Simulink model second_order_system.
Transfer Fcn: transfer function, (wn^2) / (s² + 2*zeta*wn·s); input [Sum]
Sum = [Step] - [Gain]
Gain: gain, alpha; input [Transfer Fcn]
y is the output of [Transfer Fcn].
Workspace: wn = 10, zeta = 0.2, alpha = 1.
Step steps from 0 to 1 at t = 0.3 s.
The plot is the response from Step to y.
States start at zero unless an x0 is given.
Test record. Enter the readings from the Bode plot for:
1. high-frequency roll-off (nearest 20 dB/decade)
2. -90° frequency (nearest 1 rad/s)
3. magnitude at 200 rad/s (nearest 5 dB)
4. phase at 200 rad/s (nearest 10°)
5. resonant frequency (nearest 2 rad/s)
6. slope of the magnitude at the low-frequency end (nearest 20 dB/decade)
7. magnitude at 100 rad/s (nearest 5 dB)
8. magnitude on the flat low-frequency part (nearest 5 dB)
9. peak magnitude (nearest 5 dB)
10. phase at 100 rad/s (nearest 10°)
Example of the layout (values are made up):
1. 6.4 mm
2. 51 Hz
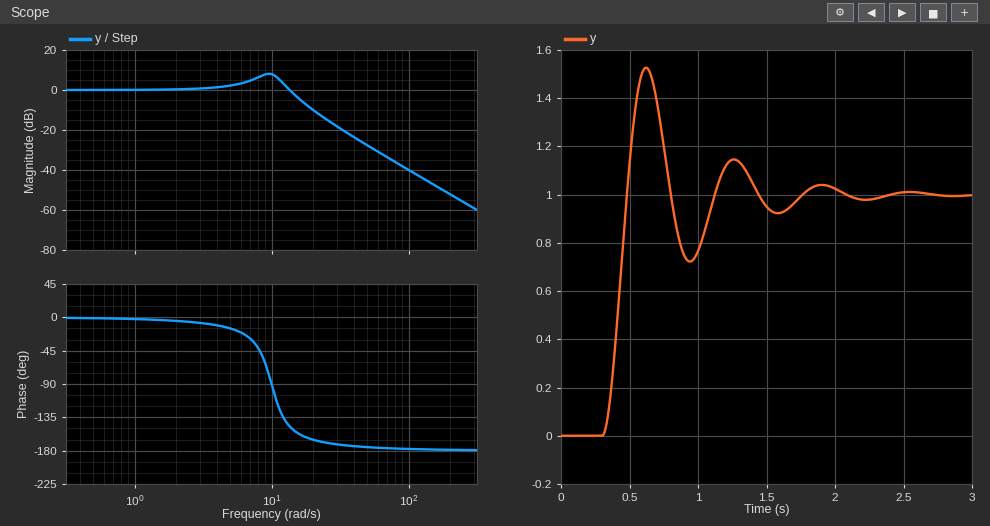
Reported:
1. -40 dB/decade
2. 10 rad/s
3. -50 dB
4. -180°
5. 10 rad/s
6. 0 dB/decade
7. -40 dB
8. 0 dB
9. 10 dB
10. -180°
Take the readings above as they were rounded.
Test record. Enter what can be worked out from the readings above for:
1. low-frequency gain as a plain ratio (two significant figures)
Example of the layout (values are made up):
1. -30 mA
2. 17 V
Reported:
1. 1.0
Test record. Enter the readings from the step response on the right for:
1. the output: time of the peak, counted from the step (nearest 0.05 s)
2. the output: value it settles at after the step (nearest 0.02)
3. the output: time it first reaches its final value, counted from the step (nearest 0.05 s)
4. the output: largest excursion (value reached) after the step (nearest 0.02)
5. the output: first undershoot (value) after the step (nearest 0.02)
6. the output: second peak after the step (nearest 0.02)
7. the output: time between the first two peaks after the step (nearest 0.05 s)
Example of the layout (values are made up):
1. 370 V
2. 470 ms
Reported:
1. 0.30 s
2. 1.00
3. 0.20 s
4. 1.52
5. 0.72
6. 1.14
7. 0.65 s
